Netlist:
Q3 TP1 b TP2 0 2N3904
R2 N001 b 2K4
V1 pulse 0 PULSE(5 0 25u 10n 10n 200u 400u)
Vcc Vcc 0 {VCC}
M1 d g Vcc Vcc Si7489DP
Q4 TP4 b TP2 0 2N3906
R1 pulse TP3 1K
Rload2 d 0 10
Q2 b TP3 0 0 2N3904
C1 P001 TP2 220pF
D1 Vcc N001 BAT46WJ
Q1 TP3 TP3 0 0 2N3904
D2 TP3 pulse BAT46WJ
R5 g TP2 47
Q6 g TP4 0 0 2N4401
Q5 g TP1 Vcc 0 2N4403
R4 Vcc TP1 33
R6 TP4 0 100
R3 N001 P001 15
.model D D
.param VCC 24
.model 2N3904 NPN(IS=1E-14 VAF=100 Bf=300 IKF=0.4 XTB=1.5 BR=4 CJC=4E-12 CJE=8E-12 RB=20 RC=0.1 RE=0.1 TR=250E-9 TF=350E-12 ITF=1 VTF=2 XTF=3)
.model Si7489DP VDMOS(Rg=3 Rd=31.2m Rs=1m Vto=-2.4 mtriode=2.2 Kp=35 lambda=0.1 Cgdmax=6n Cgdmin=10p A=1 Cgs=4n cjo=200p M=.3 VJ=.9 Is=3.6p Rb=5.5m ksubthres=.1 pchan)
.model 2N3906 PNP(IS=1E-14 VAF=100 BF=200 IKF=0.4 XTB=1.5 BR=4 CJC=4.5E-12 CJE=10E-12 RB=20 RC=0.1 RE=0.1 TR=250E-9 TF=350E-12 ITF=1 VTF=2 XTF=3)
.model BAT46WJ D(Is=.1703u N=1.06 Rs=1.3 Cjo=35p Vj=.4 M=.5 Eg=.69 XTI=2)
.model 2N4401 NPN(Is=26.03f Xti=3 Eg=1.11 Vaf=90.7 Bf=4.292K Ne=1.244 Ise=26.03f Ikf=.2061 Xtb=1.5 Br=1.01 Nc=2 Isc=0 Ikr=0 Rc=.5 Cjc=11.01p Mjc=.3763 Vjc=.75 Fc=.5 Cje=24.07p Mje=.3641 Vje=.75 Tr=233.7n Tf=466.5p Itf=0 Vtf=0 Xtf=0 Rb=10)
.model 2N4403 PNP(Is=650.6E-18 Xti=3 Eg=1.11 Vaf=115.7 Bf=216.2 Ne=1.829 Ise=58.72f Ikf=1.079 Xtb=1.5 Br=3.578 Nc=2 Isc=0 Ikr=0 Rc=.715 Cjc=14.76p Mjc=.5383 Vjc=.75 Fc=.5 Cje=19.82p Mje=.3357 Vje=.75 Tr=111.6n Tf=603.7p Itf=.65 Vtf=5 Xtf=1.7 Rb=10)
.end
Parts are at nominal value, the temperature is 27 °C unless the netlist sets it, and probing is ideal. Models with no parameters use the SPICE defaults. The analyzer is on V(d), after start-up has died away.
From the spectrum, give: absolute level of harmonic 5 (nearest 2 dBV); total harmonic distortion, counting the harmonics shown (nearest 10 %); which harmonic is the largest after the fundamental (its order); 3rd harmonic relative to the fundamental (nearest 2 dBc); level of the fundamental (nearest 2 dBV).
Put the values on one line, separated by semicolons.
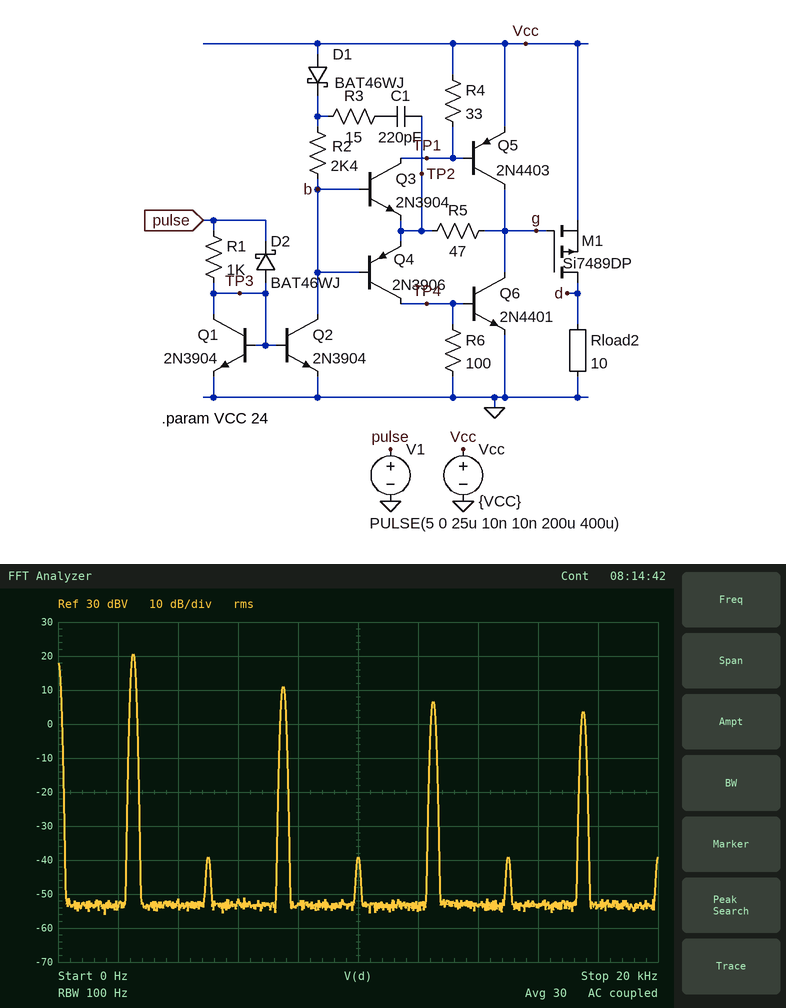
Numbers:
6 dBV; 40 %; 3; -10 dBc; 20 dBV
